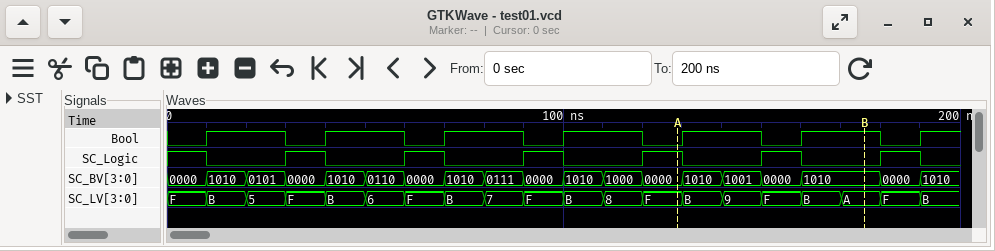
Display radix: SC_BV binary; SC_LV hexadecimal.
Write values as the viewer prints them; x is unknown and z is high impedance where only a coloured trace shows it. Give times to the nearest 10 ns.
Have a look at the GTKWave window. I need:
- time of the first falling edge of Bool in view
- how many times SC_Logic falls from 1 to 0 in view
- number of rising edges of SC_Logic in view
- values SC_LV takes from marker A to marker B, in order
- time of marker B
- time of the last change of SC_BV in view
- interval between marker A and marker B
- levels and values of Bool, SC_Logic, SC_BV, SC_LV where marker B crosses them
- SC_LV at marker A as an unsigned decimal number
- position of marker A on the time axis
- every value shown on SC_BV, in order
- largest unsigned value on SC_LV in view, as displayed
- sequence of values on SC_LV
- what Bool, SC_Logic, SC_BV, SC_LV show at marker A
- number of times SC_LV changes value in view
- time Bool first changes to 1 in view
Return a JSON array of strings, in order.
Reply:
["30 ns", "7", "6", "F, B, 9, F, B, A", "180 ns", "190 ns", "50 ns", "Bool=1, SC_Logic=0, SC_BV=1010, SC_LV=A", "15", "130 ns", "0000, 1010, 0101, 0000, 1010, 0110, 0000, 1010, 0111, 0000, 1010, 1000, 0000, 1010, 1001, 0000, 1010, 0000, 1010", "F", "F, B, 5, F, B, 6, F, B, 7, F, B, 8, F, B, 9, F, B, A, F, B", "Bool=0, SC_Logic=1, SC_BV=0000, SC_LV=F", "19", "10 ns"]
